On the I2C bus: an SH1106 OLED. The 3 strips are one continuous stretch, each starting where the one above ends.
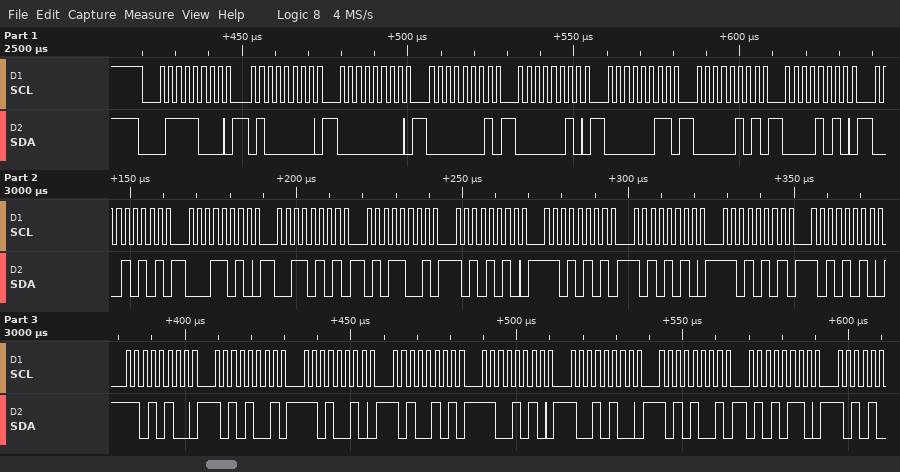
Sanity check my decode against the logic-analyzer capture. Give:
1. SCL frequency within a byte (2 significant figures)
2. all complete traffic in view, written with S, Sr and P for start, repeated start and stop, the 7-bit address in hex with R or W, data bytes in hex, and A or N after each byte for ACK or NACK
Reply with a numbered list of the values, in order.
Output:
1. 400 kHz
2. S 3CW A 40 A 00 A 01 A 02 A 03 A 05 A 0A A 15 A 1A A 35 A 59 A AA A D5 A AA A D5 A AA A D4 A A9 A D2 A A5 A CA A 94 A A9 A 56 A
